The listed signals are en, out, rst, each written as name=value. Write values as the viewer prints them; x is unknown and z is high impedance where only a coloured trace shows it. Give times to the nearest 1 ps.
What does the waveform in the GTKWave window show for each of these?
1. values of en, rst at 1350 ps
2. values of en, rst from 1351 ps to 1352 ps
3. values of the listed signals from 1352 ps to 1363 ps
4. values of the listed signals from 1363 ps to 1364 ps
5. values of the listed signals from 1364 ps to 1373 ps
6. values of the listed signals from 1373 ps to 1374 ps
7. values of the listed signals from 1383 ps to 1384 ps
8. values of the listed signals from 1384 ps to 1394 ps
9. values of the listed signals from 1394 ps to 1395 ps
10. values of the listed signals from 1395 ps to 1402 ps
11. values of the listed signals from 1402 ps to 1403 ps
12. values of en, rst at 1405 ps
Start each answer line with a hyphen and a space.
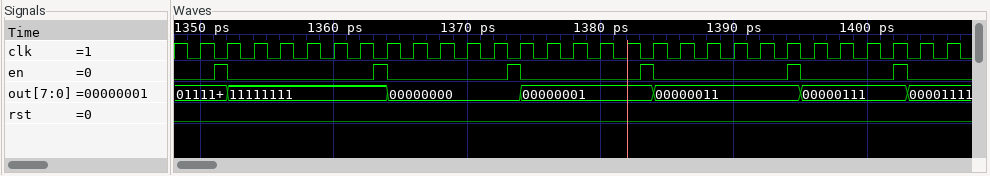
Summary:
- en=0, rst=0
- en=1, rst=0
- en=0, out=11111111, rst=0
- en=1, out=11111111, rst=0
- en=0, out=00000000, rst=0
- en=1, out=00000000, rst=0
- en=1, out=00000001, rst=0
- en=0, out=00000011, rst=0
- en=1, out=00000011, rst=0
- en=0, out=00000111, rst=0
- en=1, out=00000111, rst=0
- en=0, rst=0
